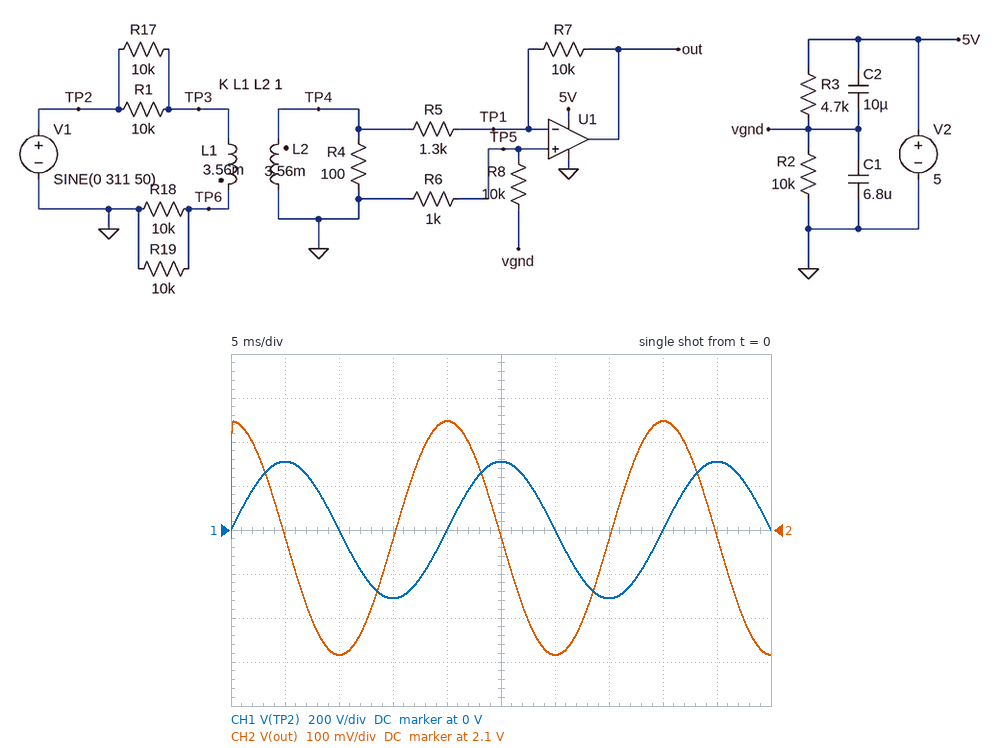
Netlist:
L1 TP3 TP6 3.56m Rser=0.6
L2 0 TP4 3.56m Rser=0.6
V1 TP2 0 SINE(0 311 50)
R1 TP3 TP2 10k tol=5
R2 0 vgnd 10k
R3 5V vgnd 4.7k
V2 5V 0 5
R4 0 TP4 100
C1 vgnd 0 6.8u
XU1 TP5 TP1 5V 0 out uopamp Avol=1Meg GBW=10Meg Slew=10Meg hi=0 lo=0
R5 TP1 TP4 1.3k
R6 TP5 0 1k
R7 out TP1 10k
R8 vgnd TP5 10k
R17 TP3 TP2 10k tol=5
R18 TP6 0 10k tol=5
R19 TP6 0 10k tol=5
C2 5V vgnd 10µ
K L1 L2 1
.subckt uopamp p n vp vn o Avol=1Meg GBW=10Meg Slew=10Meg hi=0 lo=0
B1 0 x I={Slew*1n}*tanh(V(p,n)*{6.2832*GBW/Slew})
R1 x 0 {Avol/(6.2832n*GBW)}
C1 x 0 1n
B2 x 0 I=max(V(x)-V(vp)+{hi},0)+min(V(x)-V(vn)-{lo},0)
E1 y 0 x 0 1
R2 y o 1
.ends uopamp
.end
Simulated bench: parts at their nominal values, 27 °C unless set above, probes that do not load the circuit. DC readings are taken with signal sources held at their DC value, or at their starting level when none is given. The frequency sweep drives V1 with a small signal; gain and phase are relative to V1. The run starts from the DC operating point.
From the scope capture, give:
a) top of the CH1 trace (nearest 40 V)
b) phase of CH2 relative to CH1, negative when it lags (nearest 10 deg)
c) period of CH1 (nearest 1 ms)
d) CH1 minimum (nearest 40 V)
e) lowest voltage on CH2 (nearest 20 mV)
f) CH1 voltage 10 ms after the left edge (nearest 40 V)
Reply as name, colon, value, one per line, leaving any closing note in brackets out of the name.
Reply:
top of the CH1 trace: 320 V
phase of CH2 relative to CH1, negative when it lags: 90 deg
period of CH1: 20 ms
CH1 minimum: -320 V
lowest voltage on CH2: 1.82 V
CH1 voltage 10 ms after the left edge: 0 V
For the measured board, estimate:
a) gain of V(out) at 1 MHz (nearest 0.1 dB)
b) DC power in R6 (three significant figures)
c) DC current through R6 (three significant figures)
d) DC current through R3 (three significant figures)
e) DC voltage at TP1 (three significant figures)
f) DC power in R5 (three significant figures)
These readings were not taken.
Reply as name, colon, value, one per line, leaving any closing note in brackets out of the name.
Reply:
gain of V(out) at 1 MHz: -25.2 dB
DC power in R6: 57.4 µW
DC current through R6: 240 µA
DC current through R3: 503 µA
DC voltage at TP1: 240 mV
DC power in R5: 44.1 µW
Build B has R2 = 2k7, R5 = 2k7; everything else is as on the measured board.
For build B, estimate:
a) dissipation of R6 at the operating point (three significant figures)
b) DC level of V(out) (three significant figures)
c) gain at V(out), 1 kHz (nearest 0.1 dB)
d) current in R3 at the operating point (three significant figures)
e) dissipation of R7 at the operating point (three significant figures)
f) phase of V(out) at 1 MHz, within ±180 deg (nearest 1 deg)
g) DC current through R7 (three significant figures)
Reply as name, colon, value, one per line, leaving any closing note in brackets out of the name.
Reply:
dissipation of R6 at the operating point: 20.6 µW
DC level of V(out): 675 mV
gain at V(out), 1 kHz: -41.9 dB
current in R3 at the operating point: 728 µA
dissipation of R7 at the operating point: 28.2 µW
phase of V(out) at 1 MHz, within ±180 deg: -24 deg
DC current through R7: 53.1 µA
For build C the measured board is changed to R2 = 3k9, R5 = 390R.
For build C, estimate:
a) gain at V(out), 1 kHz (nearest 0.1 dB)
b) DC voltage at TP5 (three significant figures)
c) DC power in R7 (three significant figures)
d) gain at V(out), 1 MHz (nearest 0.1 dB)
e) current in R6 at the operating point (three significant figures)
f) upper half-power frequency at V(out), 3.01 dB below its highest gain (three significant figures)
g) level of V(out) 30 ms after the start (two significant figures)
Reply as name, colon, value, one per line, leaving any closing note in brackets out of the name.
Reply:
gain at V(out), 1 kHz: -25.2 dB
DC voltage at TP5: 173 mV
DC power in R7: 1.95 mW
gain at V(out), 1 MHz: -21.4 dB
current in R6 at the operating point: 173 µA
upper half-power frequency at V(out), 3.01 dB below its highest gain: 474 kHz
level of V(out) 30 ms after the start: 3.7 V
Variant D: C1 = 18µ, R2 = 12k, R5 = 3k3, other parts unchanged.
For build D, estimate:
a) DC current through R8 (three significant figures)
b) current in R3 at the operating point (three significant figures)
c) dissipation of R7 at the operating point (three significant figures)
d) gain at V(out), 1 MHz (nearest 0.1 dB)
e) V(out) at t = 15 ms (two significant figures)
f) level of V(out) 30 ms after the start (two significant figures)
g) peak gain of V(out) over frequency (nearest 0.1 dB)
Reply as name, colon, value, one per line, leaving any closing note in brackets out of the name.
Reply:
DC current through R8: 250 µA
current in R3 at the operating point: 479 µA
dissipation of R7 at the operating point: 57.3 µW
gain at V(out), 1 MHz: -31.3 dB
V(out) at t = 15 ms: 1.0 V
level of V(out) 30 ms after the start: 900 mV
peak gain of V(out) over frequency: -30.7 dB
